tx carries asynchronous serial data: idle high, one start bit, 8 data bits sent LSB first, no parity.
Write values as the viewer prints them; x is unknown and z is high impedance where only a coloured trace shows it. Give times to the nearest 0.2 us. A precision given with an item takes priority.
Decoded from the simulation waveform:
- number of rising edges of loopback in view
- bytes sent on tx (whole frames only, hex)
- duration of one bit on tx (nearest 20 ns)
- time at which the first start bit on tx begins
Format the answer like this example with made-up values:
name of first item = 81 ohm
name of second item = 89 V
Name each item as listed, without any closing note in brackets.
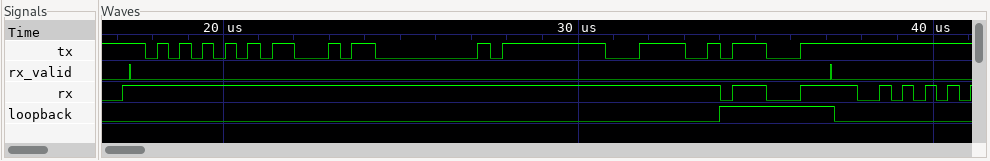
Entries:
number of rising edges of loopback in view = 1
bytes sent on tx = 55, A3, 00, FF, 3C, C7
duration of one bit on tx = 320 ns
time at which the first start bit on tx begins = 17.8 us
